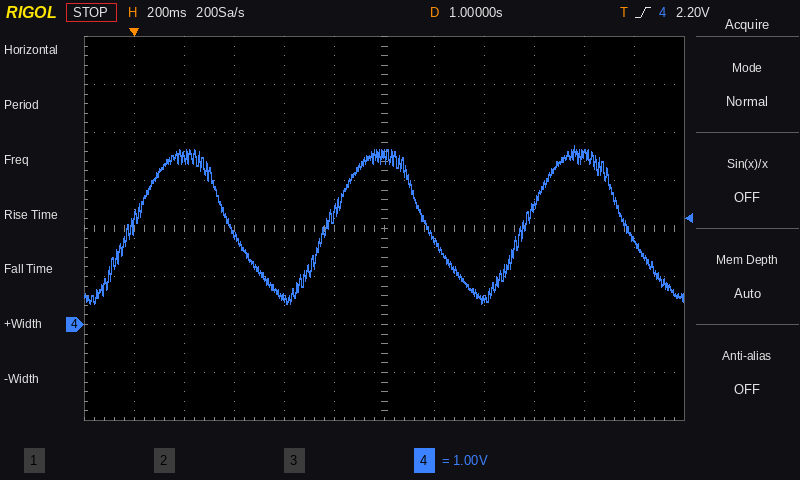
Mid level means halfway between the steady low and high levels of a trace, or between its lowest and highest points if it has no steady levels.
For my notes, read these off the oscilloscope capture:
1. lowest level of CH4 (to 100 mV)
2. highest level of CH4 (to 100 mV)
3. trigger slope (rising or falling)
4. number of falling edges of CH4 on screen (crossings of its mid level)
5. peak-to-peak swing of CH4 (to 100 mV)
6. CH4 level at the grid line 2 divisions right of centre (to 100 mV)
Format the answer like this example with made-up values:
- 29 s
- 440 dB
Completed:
- 400 mV
- 3.7 V
- rising
- 3
- 3.3 V
- 500 mV
